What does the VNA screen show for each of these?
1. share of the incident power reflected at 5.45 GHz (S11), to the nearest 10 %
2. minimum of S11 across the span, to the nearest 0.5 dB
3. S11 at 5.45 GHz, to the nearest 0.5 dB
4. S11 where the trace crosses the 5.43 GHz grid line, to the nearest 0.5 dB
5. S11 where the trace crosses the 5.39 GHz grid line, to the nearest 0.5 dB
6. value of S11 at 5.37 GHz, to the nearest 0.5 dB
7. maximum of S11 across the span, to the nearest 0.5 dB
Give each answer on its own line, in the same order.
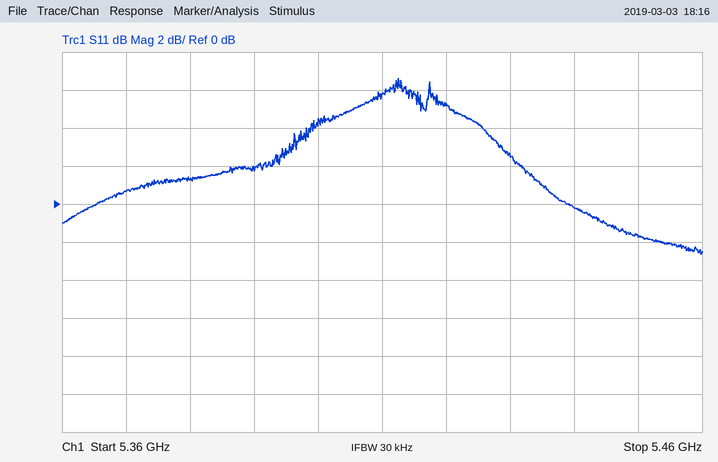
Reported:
70 %
-2.5 dB
-1.5 dB
2.5 dB
2.0 dB
0.5 dB
6.5 dB
